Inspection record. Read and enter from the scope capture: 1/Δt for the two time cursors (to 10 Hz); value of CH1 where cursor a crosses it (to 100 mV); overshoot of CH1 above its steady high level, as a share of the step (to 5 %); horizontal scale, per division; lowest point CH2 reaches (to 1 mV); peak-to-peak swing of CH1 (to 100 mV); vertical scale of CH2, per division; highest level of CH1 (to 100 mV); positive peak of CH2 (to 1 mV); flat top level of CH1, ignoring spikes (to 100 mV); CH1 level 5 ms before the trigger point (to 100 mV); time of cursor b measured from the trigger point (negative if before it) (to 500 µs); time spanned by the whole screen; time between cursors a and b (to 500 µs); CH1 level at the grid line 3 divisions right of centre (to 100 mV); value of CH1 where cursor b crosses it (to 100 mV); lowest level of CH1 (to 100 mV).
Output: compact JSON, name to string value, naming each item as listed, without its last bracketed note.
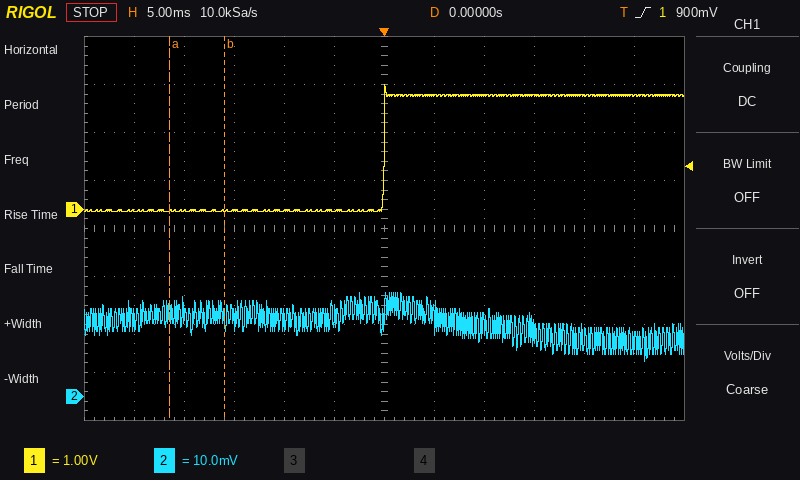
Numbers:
{"1/Δt for the two time cursors": "180 Hz", "value of CH1 where cursor a crosses it": "0.0 V", "overshoot of CH1 above its steady high level, as a share of the step": "10 %", "horizontal scale, per division": "5 ms", "lowest point CH2 reaches": "7 mV", "peak-to-peak swing of CH1": "2.6 V", "vertical scale of CH2, per division": "10 mV", "highest level of CH1": "2.6 V", "positive peak of CH2": "22 mV", "flat top level of CH1, ignoring spikes": "2.4 V", "CH1 level 5 ms before the trigger point": "0.0 V", "time of cursor b measured from the trigger point (negative if before it)": "-16.0 ms", "time spanned by the whole screen": "60 ms", "time between cursors a and b": "5.5 ms", "CH1 level at the grid line 3 divisions right of centre": "2.4 V", "value of CH1 where cursor b crosses it": "0.0 V", "lowest level of CH1": "0.0 V"}
